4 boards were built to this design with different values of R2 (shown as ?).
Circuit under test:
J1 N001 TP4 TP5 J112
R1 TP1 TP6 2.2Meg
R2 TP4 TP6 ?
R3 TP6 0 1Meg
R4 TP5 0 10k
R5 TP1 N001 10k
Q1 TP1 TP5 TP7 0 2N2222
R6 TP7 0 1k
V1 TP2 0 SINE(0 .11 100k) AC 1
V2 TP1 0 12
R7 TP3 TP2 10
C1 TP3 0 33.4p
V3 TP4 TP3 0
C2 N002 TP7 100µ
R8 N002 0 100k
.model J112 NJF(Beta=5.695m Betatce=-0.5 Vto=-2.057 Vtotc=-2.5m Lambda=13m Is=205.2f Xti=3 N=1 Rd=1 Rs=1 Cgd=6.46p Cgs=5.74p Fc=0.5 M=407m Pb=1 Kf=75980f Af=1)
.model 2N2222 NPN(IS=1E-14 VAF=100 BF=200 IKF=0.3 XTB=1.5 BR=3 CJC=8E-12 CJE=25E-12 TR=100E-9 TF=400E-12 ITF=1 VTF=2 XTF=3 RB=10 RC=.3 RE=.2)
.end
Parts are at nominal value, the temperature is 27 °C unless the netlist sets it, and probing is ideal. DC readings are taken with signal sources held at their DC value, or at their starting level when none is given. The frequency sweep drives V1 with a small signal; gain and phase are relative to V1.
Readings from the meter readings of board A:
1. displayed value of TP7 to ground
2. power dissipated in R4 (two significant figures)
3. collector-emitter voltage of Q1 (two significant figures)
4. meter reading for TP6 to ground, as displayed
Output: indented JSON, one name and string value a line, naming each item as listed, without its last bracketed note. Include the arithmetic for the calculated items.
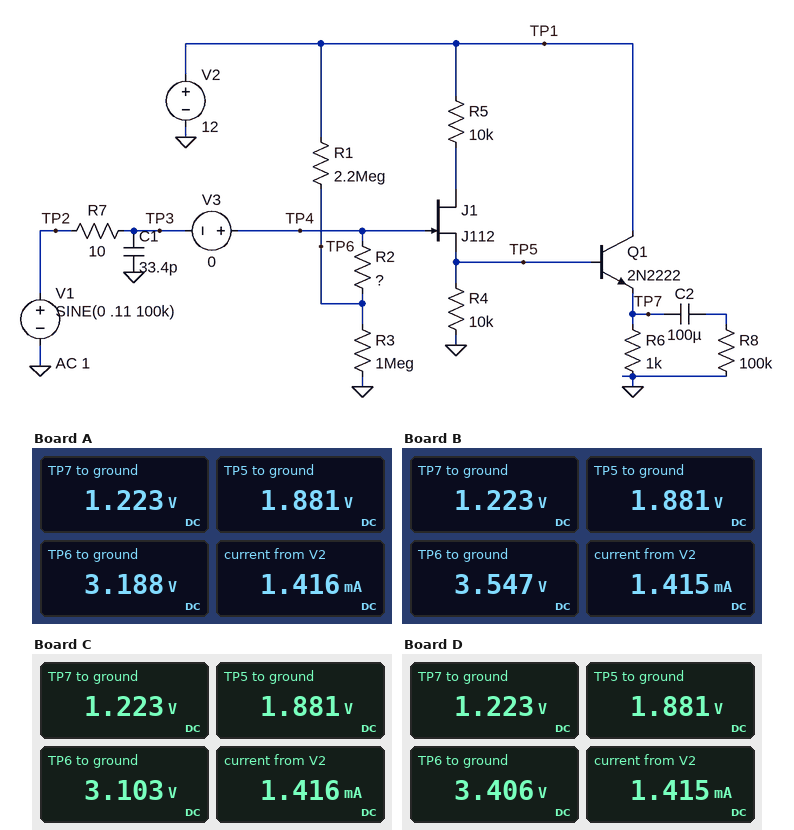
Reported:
{
  "displayed value of TP7 to ground": "1.223 V",
  "power dissipated in R4": "(1.881 V)^2 / 10 kΩ = 350 µW",
  "collector-emitter voltage of Q1": "12 V - 1.223 V = 11 V",
  "meter reading for TP6 to ground, as displayed": "3.188 V"
}
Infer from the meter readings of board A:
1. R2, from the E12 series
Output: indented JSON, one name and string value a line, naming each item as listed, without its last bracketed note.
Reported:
{
  "R2, from the E12 series": "3.9 MΩ"
}
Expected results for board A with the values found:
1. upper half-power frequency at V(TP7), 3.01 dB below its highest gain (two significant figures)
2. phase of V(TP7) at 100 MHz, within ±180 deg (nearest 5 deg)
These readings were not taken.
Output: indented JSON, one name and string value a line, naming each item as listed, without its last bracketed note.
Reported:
{
  "upper half-power frequency at V(TP7), 3.01 dB below its highest gain": "56 MHz",
  "phase of V(TP7) at 100 MHz, within ±180 deg": "-30 deg"
}
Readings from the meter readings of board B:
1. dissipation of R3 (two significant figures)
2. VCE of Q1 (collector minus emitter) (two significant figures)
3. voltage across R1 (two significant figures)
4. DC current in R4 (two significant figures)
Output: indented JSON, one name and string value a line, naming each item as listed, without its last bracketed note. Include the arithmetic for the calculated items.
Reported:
{
  "dissipation of R3": "(3.547 V)^2 / 1 MΩ = 13 µW",
  "VCE of Q1 (collector minus emitter)": "12 V - 1.223 V = 11 V",
  "voltage across R1": "12 V - 3.547 V = 8.5 V",
  "DC current in R4": "(1.881 V) / 10 kΩ = 190 µA"
}
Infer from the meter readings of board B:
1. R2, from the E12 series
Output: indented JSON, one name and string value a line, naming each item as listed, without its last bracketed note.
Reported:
{
  "R2, from the E12 series": "12 MΩ"
}
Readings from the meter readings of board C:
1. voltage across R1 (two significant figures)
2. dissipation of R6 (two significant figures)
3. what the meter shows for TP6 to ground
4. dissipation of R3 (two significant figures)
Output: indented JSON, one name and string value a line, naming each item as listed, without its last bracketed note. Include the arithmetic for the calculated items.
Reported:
{
  "voltage across R1": "12 V - 3.103 V = 8.9 V",
  "dissipation of R6": "(1.223 V)^2 / 1 kΩ = 1.5 mW",
  "what the meter shows for TP6 to ground": "3.103 V",
  "dissipation of R3": "(3.103 V)^2 / 1 MΩ = 9.6 µW"
}
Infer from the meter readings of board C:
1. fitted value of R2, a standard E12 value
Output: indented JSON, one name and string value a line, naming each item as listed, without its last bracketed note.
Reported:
{
  "fitted value of R2, a standard E12 value": "3.3 MΩ"
}
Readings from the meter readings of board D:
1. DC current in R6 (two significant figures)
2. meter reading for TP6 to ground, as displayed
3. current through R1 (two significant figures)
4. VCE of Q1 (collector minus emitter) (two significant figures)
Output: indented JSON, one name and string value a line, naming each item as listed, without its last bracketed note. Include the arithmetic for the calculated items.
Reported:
{
  "DC current in R6": "(1.223 V) / 1 kΩ = 1.2 mA",
  "meter reading for TP6 to ground, as displayed": "3.406 V",
  "current through R1": "(12 V - 3.406 V) / 2.2 MΩ = 3.9 µA",
  "VCE of Q1 (collector minus emitter)": "12 V - 1.223 V = 11 V"
}
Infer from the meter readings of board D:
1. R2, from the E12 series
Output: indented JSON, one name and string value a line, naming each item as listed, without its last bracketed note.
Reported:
{
  "R2, from the E12 series": "6.8 MΩ"
}
